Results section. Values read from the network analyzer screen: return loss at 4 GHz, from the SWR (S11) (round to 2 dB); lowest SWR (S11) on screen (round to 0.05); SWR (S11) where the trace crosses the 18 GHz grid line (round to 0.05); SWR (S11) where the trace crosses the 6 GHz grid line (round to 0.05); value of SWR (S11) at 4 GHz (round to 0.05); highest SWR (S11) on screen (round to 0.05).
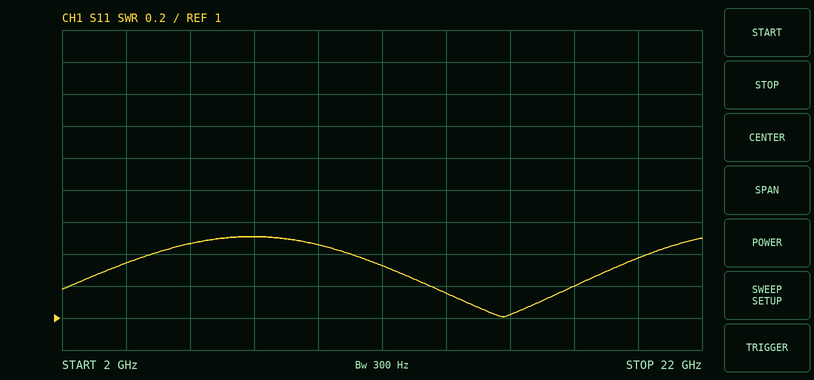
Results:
16 dB
1.00
1.20
1.45
1.35
1.50
